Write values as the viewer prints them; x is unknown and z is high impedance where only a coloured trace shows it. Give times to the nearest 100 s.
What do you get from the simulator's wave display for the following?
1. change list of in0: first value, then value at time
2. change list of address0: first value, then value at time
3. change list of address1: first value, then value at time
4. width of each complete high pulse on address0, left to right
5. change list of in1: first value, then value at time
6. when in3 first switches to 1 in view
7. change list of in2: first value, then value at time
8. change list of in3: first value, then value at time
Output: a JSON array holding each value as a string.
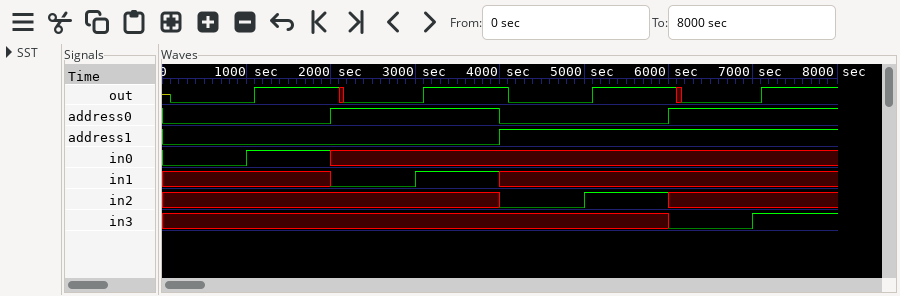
["0, 1 at 1000 s, x at 2000 s", "0, 1 at 2000 s, 0 at 4000 s, 1 at 6000 s", "0, 1 at 4000 s", "2000 s", "x, 0 at 2000 s, 1 at 3000 s, x at 4000 s", "7000 s", "x, 0 at 4000 s, 1 at 5000 s, x at 6000 s", "x, 0 at 6000 s, 1 at 7000 s"]
